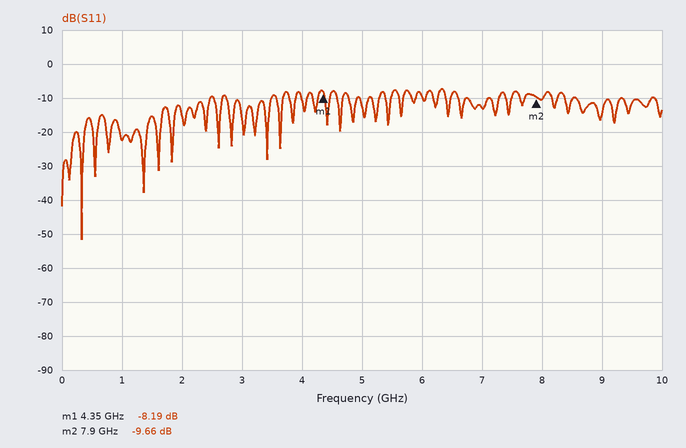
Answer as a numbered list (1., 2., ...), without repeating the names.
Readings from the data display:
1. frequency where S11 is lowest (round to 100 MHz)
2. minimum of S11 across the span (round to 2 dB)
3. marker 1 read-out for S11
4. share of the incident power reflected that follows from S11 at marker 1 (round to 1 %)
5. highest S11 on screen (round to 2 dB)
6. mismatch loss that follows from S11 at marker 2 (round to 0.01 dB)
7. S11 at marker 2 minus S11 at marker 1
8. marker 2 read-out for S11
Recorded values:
1. 300 MHz
2. -52 dB
3. -8.19 dB
4. 15 %
5. -8 dB
6. 0.50 dB
7. -1.47 dB
8. -9.66 dB
